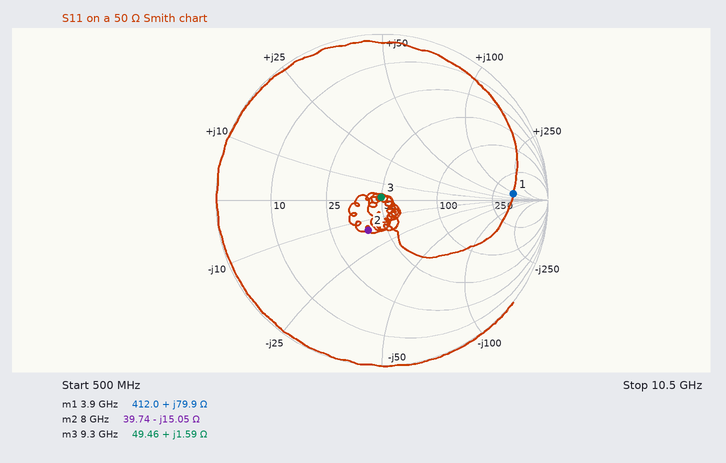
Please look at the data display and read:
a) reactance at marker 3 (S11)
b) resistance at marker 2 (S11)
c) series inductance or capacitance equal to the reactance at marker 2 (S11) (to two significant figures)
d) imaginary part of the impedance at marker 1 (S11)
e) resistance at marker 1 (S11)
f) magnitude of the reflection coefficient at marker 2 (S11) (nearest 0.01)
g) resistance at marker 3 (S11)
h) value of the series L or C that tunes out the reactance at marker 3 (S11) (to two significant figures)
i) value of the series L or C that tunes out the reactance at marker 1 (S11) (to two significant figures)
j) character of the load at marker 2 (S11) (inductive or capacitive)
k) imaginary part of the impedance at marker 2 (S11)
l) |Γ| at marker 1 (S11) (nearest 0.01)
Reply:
+1.59 Ω
39.74 Ω
1.3 pF
+79.9 Ω
412.0 Ω
0.20
49.46 Ω
11 pF
510 fF
capacitive
-15.05 Ω
0.79
